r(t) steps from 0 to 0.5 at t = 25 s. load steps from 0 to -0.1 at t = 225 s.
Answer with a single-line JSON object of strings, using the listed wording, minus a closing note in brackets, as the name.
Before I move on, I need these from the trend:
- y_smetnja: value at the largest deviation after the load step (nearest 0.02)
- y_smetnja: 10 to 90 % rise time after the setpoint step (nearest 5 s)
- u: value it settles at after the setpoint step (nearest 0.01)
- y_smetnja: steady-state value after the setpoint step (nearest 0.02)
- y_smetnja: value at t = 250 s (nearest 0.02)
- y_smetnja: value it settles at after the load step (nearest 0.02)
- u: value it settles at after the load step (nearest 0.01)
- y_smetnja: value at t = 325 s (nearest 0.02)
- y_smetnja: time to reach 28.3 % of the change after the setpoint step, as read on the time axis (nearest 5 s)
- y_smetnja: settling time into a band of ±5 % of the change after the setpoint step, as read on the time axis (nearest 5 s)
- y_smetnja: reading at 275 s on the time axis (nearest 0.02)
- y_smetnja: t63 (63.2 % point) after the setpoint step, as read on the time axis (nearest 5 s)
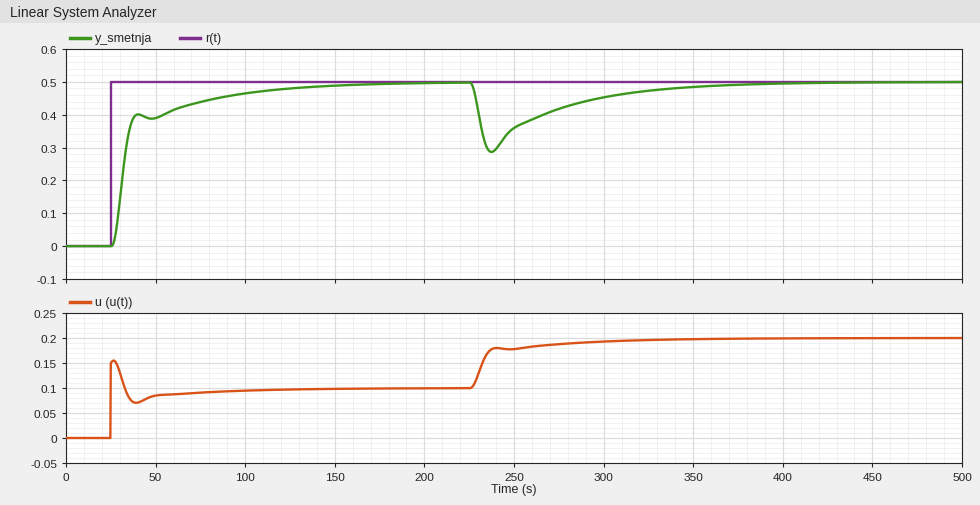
{"y_smetnja: value at the largest deviation after the load step": "0.28", "y_smetnja: 10 to 90 % rise time after the setpoint step": "55 s", "u: value it settles at after the setpoint step": "0.10", "y_smetnja: steady-state value after the setpoint step": "0.50", "y_smetnja: value at t = 250 s": "0.36", "y_smetnja: value it settles at after the load step": "0.50", "u: value it settles at after the load step": "0.20", "y_smetnja: value at t = 325 s": "0.48", "y_smetnja: time to reach 28.3 % of the change after the setpoint step, as read on the time axis": "30 s", "y_smetnja: settling time into a band of ±5 % of the change after the setpoint step, as read on the time axis": "115 s", "y_smetnja: reading at 275 s on the time axis": "0.42", "y_smetnja: t63 (63.2 % point) after the setpoint step, as read on the time axis": "35 s"}
